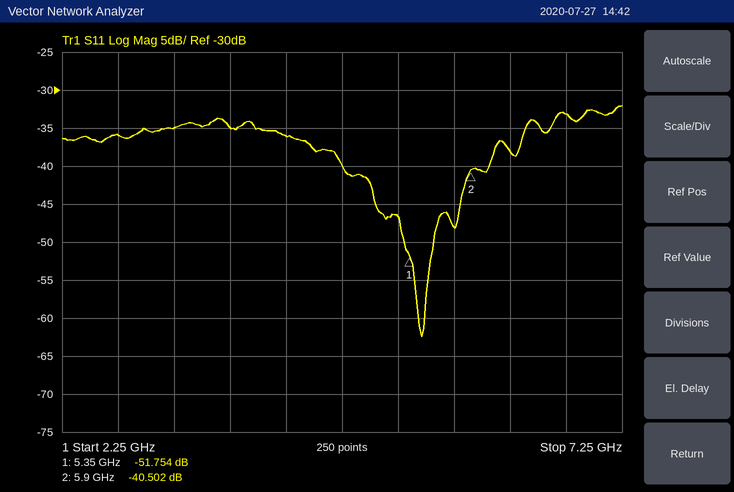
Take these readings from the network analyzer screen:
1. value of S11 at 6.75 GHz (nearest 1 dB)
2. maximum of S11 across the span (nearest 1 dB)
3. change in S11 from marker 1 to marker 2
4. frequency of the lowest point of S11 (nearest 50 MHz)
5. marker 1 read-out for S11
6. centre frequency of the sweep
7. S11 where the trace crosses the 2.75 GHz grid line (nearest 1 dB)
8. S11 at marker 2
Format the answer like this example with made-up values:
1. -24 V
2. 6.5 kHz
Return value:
1. -33 dB
2. -32 dB
3. 11.252 dB
4. 5.45 GHz
5. -51.754 dB
6. 4.75 GHz
7. -36 dB
8. -40.502 dB
